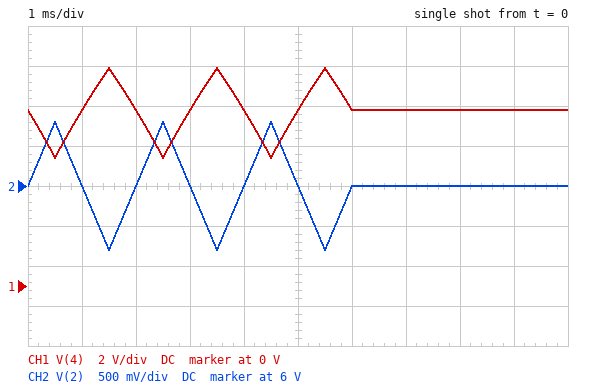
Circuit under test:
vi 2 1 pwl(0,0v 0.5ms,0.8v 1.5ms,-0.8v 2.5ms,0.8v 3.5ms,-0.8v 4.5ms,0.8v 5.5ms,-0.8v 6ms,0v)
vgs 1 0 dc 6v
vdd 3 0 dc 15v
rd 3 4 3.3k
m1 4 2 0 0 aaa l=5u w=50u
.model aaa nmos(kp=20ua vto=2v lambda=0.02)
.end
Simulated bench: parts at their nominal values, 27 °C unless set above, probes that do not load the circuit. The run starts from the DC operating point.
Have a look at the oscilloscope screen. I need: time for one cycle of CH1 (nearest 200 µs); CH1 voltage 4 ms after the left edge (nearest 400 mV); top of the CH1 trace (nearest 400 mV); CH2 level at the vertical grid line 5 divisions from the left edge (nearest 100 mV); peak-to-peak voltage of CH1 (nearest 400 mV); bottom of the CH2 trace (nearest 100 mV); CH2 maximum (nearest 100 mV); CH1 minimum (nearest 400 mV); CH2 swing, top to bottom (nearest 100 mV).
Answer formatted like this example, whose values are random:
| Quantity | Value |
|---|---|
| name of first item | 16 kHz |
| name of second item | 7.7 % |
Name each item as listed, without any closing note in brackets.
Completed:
| Quantity | Value |
|---|---|
| time for one cycle of CH1 | 2.0 ms |
| CH1 voltage 4 ms after the left edge | 8.8 V |
| top of the CH1 trace | 10.8 V |
| CH2 level at the vertical grid line 5 divisions from the left edge | 6.0 V |
| peak-to-peak voltage of CH1 | 4.4 V |
| bottom of the CH2 trace | 5.2 V |
| CH2 maximum | 6.8 V |
| CH1 minimum | 6.4 V |
| CH2 swing, top to bottom | 1.6 V |
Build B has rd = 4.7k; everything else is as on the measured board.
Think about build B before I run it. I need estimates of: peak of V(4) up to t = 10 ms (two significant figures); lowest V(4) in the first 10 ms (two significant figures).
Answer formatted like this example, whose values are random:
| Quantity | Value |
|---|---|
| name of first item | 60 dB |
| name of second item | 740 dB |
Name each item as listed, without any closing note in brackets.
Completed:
| Quantity | Value |
|---|---|
| peak of V(4) up to t = 10 ms | 9.3 V |
| lowest V(4) in the first 10 ms | 3.8 V |
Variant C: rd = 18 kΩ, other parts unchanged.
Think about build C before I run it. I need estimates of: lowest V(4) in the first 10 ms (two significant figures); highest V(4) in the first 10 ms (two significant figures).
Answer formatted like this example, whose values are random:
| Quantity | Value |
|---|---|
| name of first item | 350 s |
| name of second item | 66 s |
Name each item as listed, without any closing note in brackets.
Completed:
| Quantity | Value |
|---|---|
| lowest V(4) in the first 10 ms | 880 mV |
| highest V(4) in the first 10 ms | 1.5 V |
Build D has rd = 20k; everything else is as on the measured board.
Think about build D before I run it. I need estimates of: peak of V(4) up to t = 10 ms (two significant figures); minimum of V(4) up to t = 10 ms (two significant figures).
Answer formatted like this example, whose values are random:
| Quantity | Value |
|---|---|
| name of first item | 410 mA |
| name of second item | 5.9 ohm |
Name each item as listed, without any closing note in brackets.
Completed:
| Quantity | Value |
|---|---|
| peak of V(4) up to t = 10 ms | 1.3 V |
| minimum of V(4) up to t = 10 ms | 790 mV |
